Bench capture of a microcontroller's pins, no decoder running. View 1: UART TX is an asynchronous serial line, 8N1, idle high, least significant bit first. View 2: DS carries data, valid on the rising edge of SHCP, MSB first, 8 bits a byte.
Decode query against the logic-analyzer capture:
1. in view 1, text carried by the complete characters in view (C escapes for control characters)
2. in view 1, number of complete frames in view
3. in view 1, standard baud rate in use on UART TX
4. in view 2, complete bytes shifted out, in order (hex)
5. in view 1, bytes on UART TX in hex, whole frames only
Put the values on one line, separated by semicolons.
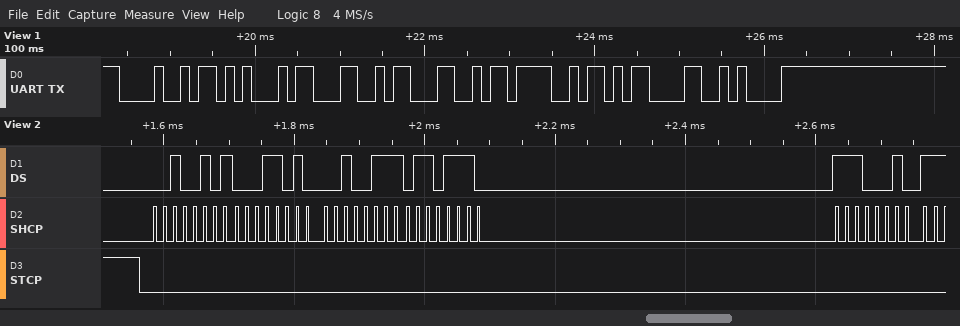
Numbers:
"HELLO\r\n"; 7; 9600 baud; 25 1A 27 6E E2; 48 45 4C 4C 4F 0D 0A
